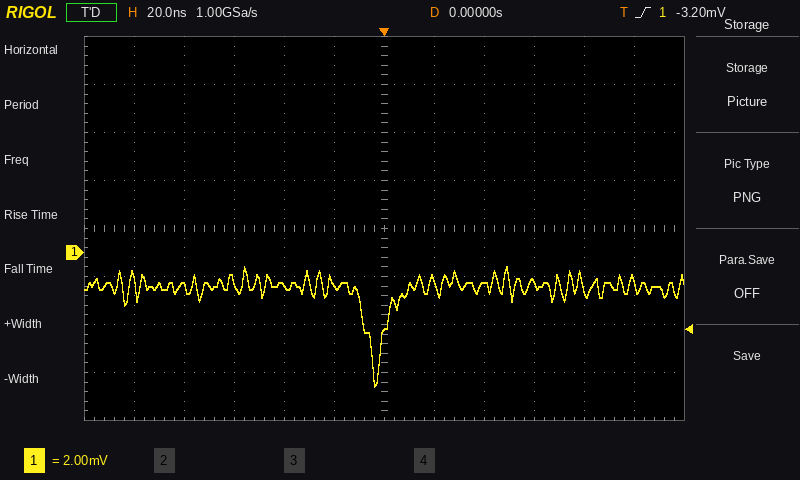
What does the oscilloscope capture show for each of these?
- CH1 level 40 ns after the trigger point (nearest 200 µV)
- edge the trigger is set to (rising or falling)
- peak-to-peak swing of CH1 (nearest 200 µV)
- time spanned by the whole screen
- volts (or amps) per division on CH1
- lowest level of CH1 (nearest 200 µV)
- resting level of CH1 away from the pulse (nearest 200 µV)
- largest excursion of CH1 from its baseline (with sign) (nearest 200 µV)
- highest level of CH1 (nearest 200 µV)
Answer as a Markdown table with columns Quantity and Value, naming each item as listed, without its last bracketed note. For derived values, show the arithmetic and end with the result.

| Quantity | Value |
|---|---|
| CH1 level 40 ns after the trigger point | -1.2 mV |
| edge the trigger is set to | rising |
| peak-to-peak swing of CH1 | -600 µV − (-5.6 mV) = 5.0 mV |
| time spanned by the whole screen | 240 ns |
| volts (or amps) per division on CH1 | 2 mV |
| lowest level of CH1 | -5.6 mV |
| resting level of CH1 away from the pulse | -1.4 mV |
| largest excursion of CH1 from its baseline (with sign) | -5.6 mV − (-1.4 mV) = -4.2 mV |
| highest level of CH1 | -600 µV |
